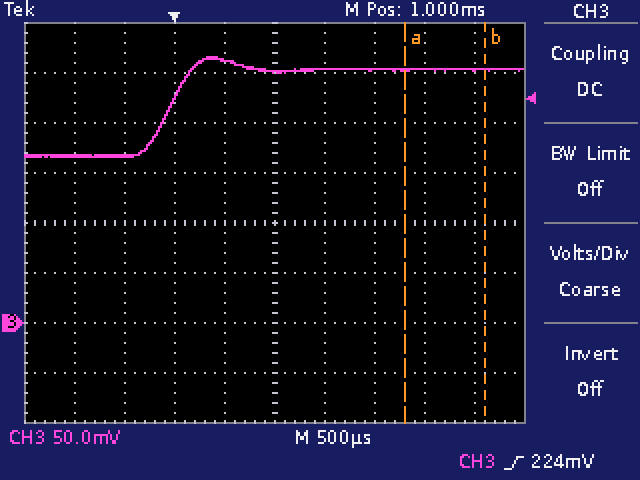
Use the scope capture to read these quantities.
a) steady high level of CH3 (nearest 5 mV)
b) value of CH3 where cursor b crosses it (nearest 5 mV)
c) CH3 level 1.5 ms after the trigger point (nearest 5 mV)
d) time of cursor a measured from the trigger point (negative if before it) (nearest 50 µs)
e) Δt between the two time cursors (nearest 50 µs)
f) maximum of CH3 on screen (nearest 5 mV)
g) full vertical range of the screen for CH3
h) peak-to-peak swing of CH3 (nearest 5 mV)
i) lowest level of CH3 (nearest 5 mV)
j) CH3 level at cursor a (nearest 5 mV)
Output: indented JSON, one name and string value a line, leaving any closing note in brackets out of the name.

{
  "steady high level of CH3": "255 mV",
  "value of CH3 where cursor b crosses it": "255 mV",
  "CH3 level 1.5 ms after the trigger point": "255 mV",
  "time of cursor a measured from the trigger point (negative if before it)": "+2.30 ms",
  "Δt between the two time cursors": "800 µs",
  "maximum of CH3 on screen": "265 mV",
  "full vertical range of the screen for CH3": "400 mV",
  "peak-to-peak swing of CH3": "100 mV",
  "lowest level of CH3": "165 mV",
  "CH3 level at cursor a": "255 mV"
}
